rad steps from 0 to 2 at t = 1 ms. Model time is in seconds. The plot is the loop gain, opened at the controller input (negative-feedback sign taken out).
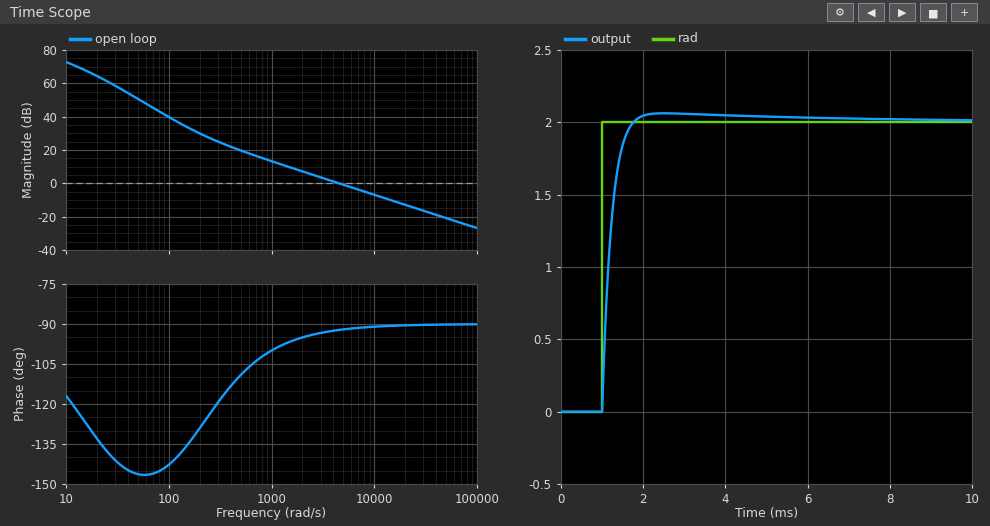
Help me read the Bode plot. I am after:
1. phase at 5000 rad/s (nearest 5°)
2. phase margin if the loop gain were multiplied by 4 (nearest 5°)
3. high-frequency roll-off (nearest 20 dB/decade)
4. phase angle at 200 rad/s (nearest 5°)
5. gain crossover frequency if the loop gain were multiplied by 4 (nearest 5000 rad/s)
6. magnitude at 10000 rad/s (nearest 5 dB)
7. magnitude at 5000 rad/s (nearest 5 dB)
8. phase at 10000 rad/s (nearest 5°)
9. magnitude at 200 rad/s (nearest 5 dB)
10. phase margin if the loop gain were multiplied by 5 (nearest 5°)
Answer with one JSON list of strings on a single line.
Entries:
["-90°", "90°", "-20 dB/decade", "-130°", "20000 rad/s", "-5 dB", "0 dB", "-90°", "30 dB", "90°"]
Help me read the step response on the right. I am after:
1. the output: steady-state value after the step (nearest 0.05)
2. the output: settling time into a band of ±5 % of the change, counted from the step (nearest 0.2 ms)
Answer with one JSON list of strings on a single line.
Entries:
["2.00", "0.6 ms"]
